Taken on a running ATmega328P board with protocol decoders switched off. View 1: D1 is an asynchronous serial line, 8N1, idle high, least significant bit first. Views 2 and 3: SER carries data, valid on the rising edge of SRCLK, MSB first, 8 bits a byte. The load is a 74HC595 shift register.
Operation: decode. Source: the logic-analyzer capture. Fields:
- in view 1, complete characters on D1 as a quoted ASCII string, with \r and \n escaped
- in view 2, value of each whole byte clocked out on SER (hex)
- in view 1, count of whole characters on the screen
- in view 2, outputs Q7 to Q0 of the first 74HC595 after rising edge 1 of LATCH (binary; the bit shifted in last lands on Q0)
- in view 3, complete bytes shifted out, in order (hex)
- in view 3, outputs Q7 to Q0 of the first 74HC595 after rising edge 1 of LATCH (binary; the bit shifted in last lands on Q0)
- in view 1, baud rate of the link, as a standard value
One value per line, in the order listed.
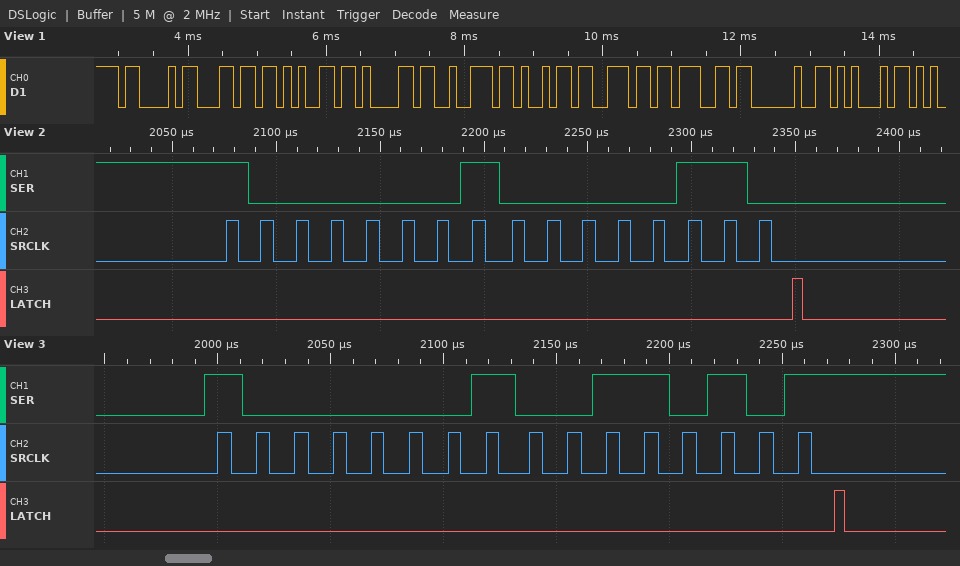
"Clearing E"
81 06
10
00000110
81 35
00110101
9600 baud
